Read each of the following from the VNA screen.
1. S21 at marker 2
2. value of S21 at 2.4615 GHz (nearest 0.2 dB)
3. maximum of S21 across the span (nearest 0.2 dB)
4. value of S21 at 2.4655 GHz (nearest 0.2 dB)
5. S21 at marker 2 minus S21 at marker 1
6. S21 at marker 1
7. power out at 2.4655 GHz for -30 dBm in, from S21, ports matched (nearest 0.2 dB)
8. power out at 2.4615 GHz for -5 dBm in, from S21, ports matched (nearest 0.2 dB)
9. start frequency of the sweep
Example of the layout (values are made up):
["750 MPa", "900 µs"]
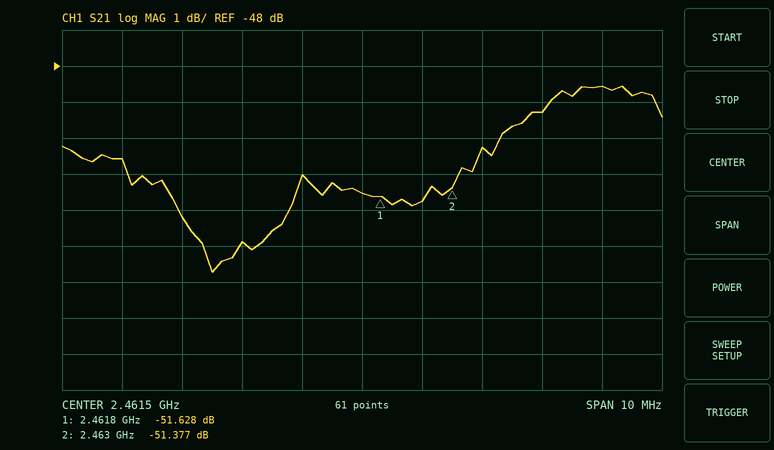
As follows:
["-51.377 dB", "-51.6 dB", "-48.6 dB", "-48.6 dB", "0.251 dB", "-51.628 dB", "-78.6 dBm", "-56.6 dBm", "2.4565 GHz"]
